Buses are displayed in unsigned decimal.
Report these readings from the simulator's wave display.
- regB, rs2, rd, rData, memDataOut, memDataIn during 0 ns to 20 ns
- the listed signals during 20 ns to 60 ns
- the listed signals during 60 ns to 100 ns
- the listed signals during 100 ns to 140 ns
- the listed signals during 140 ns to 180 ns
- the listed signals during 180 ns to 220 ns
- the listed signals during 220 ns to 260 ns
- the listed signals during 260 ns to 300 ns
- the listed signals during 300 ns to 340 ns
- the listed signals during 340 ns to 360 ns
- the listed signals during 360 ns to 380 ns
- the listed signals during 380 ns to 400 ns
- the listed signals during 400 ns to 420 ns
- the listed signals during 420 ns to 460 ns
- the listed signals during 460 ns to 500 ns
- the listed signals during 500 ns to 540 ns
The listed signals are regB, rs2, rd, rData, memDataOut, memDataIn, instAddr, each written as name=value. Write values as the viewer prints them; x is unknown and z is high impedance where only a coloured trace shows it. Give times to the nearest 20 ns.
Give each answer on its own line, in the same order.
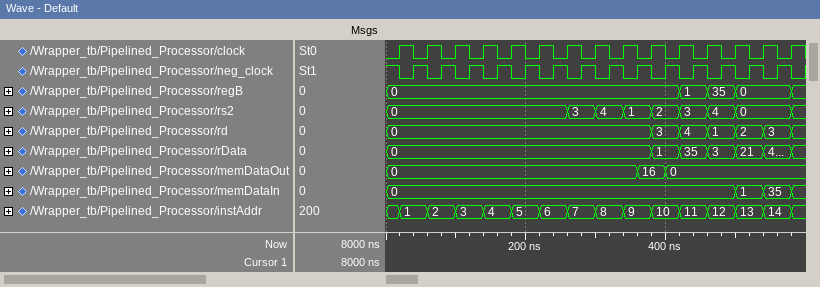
regB=0, rs2=0, rd=0, rData=0, memDataOut=0, memDataIn=0
regB=0, rs2=0, rd=0, rData=0, memDataOut=0, memDataIn=0, instAddr=1
regB=0, rs2=0, rd=0, rData=0, memDataOut=0, memDataIn=0, instAddr=2
regB=0, rs2=0, rd=0, rData=0, memDataOut=0, memDataIn=0, instAddr=3
regB=0, rs2=0, rd=0, rData=0, memDataOut=0, memDataIn=0, instAddr=4
regB=0, rs2=0, rd=0, rData=0, memDataOut=0, memDataIn=0, instAddr=5
regB=0, rs2=0, rd=0, rData=0, memDataOut=0, memDataIn=0, instAddr=6
regB=0, rs2=3, rd=0, rData=0, memDataOut=0, memDataIn=0, instAddr=7
regB=0, rs2=4, rd=0, rData=0, memDataOut=0, memDataIn=0, instAddr=8
regB=0, rs2=1, rd=0, rData=0, memDataOut=0, memDataIn=0, instAddr=9
regB=0, rs2=1, rd=0, rData=0, memDataOut=16, memDataIn=0, instAddr=9
regB=0, rs2=2, rd=3, rData=1, memDataOut=16, memDataIn=0, instAddr=10
regB=0, rs2=2, rd=3, rData=1, memDataOut=0, memDataIn=0, instAddr=10
regB=1, rs2=3, rd=4, rData=35, memDataOut=0, memDataIn=0, instAddr=11
regB=35, rs2=4, rd=1, rData=3, memDataOut=0, memDataIn=0, instAddr=12
regB=0, rs2=0, rd=2, rData=21, memDataOut=0, memDataIn=1, instAddr=13
